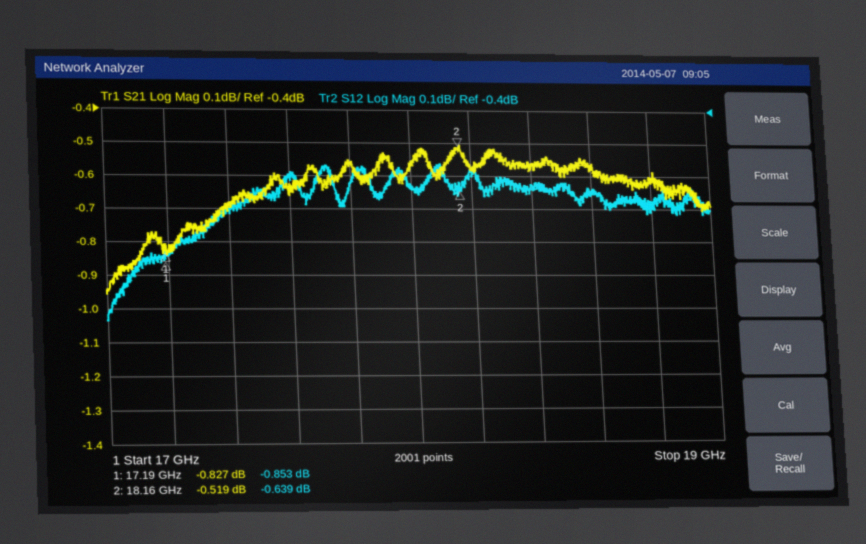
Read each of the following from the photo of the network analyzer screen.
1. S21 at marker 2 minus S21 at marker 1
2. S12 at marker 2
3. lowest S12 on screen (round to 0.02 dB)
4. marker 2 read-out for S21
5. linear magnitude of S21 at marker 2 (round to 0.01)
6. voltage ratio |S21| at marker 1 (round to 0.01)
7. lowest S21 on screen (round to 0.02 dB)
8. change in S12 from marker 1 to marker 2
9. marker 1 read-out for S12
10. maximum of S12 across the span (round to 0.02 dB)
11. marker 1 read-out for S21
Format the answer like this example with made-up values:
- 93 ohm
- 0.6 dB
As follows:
- 0.308 dB
- -0.639 dB
- -1.04 dB
- -0.519 dB
- 0.94
- 0.91
- -0.96 dB
- 0.214 dB
- -0.853 dB
- -0.56 dB
- -0.827 dB
